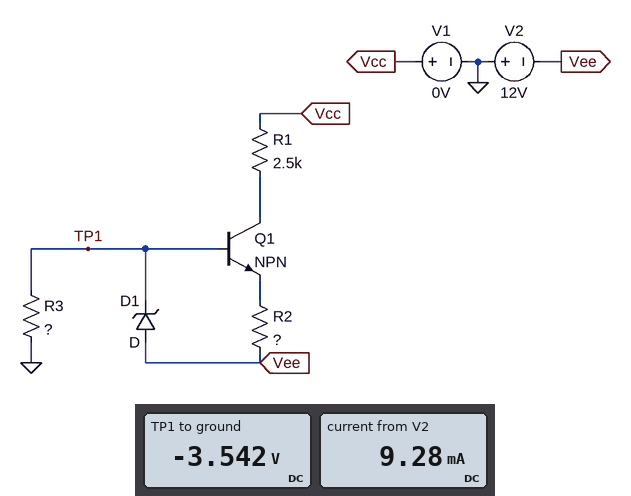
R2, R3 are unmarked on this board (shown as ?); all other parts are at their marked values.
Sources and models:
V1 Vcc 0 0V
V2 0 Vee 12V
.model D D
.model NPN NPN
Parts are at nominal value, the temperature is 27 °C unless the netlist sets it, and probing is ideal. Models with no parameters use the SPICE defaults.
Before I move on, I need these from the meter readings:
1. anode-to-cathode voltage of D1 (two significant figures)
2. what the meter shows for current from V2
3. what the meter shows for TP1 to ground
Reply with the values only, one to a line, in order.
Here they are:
-8.5 V
9.28 mA
-3.542 V
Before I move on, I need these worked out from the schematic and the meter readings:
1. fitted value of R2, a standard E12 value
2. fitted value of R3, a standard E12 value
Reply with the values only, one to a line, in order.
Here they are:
820 Ω
470 Ω
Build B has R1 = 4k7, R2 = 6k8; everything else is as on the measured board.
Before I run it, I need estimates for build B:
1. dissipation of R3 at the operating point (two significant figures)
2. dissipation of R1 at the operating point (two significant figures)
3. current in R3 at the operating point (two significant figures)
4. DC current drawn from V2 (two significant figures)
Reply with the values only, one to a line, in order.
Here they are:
750 µW
400 µW
1.3 mA
1.6 mA
